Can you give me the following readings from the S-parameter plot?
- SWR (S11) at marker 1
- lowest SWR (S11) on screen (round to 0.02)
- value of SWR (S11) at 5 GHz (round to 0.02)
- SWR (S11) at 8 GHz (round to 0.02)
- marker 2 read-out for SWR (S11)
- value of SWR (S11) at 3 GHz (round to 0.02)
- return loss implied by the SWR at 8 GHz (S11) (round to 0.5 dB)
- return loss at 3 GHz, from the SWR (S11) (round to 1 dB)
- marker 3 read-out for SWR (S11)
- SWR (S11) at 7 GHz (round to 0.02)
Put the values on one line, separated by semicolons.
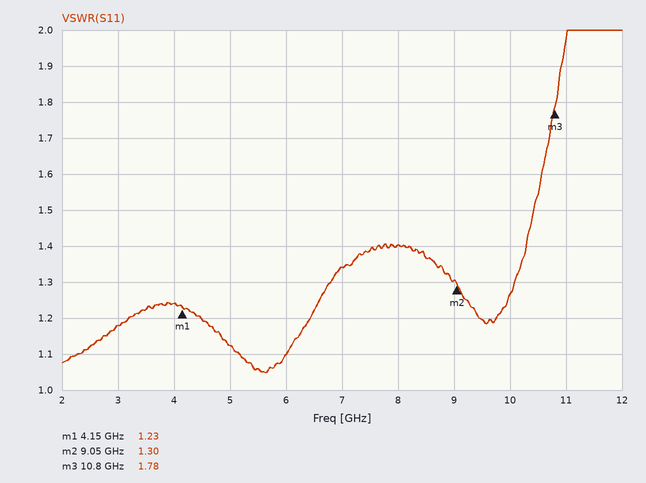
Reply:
1.23; 1.04; 1.12; 1.40; 1.30; 1.18; 15.5 dB; 22 dB; 1.78; 1.34
